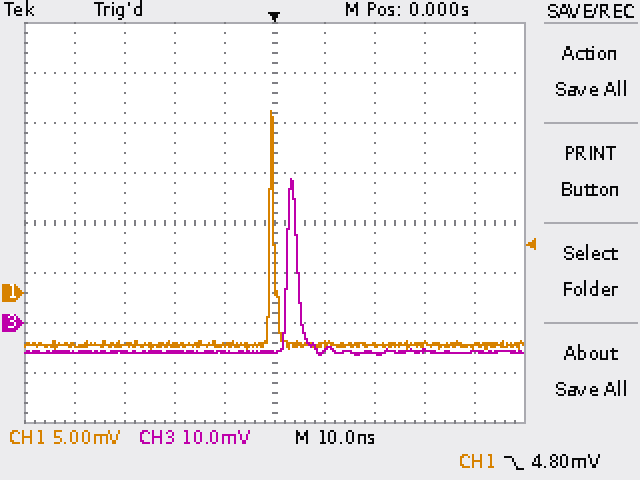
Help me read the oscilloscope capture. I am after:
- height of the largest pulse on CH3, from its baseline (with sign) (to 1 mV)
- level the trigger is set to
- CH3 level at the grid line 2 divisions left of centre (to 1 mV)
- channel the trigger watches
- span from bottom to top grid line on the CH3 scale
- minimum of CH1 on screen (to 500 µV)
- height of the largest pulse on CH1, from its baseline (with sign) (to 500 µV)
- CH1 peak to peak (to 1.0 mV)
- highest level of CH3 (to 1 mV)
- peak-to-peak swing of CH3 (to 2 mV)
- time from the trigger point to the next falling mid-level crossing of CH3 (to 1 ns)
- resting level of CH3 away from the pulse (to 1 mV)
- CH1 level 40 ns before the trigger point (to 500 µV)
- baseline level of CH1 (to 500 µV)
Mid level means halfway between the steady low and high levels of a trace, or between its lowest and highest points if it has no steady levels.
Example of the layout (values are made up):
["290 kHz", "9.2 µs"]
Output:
["+35 mV", "4.80 mV", "-6 mV", "CH1", "80 mV", "-5.5 mV", "+23.5 mV", "24.0 mV", "29 mV", "36 mV", "5 ns", "-6 mV", "-5.0 mV", "-5.0 mV"]
